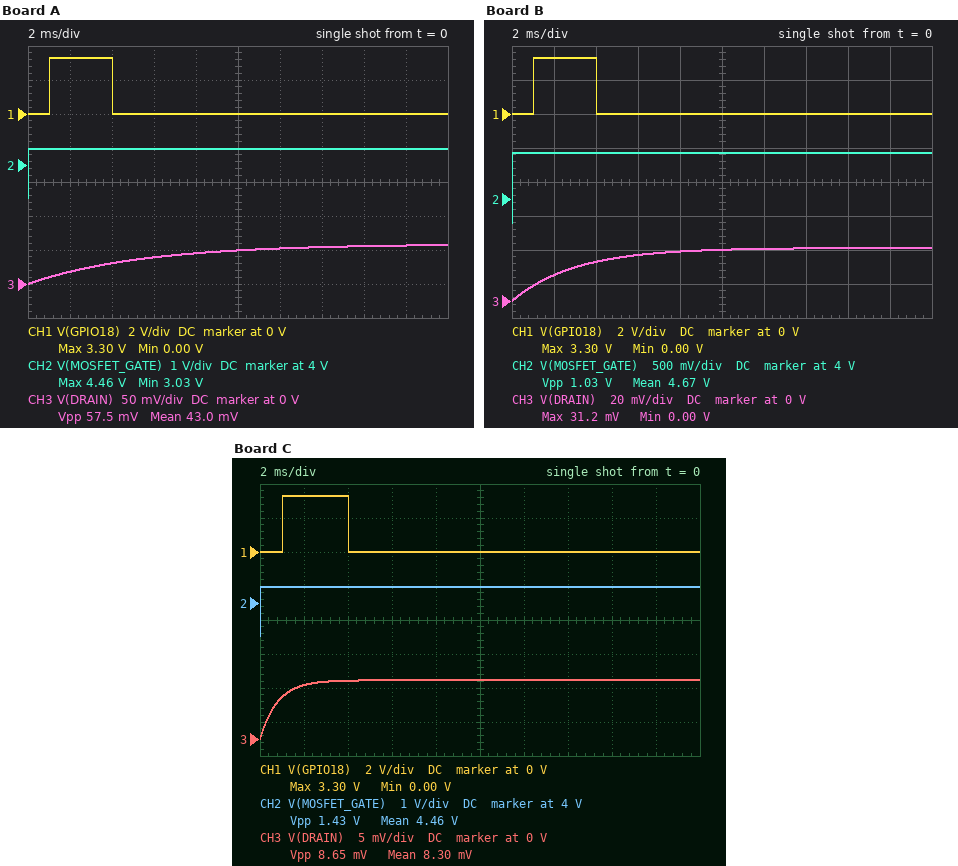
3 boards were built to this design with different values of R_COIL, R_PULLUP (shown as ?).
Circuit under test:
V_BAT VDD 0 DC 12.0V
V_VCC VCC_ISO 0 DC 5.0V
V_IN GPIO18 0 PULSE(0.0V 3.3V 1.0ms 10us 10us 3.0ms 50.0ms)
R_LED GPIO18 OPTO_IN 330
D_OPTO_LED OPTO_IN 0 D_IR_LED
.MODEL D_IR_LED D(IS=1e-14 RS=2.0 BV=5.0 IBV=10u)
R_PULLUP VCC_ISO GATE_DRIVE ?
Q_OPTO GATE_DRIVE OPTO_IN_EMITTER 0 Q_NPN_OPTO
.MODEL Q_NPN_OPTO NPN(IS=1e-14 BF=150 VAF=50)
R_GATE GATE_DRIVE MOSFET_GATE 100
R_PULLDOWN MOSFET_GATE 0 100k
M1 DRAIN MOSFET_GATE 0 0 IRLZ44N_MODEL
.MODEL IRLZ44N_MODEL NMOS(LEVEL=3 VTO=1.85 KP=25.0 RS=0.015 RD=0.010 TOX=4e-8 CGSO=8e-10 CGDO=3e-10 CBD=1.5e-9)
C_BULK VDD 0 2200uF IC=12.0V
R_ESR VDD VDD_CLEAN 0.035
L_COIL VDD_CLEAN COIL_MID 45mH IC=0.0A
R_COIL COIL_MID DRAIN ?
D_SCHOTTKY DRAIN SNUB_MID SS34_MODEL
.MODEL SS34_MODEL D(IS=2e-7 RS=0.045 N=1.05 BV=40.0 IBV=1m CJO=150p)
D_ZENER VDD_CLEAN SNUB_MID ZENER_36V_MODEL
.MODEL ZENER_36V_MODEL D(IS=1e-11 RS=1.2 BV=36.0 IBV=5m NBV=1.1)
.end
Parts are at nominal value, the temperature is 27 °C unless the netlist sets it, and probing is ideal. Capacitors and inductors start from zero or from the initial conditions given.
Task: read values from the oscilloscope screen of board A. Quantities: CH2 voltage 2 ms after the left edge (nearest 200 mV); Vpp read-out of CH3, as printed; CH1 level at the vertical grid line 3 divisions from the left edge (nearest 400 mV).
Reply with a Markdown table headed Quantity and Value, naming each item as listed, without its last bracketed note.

| Quantity | Value |
|---|---|
| CH2 voltage 2 ms after the left edge | 4.4 V |
| Vpp read-out of CH3, as printed | 57.5 mV |
| CH1 level at the vertical grid line 3 divisions from the left edge | 0 V |
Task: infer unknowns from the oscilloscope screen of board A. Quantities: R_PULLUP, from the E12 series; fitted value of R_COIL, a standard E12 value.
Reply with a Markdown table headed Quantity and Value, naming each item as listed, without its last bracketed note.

| Quantity | Value |
|---|---|
| R_PULLUP, from the E12 series | 12 kΩ |
| fitted value of R_COIL, a standard E12 value | 8.2 Ω |
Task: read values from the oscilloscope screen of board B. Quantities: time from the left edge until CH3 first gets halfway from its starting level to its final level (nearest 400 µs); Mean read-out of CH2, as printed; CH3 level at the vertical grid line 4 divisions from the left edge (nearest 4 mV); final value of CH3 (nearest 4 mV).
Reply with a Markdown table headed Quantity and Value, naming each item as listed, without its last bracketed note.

| Quantity | Value |
|---|---|
| time from the left edge until CH3 first gets halfway from its starting level to its final level | 2.0 ms |
| Mean read-out of CH2, as printed | 4.67 V |
| CH3 level at the vertical grid line 4 divisions from the left edge | 28 mV |
| final value of CH3 | 32 mV |
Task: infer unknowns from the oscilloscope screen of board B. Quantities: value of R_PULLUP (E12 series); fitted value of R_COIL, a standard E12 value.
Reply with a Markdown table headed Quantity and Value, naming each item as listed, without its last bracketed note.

| Quantity | Value |
|---|---|
| value of R_PULLUP | 6.8 kΩ |
| fitted value of R_COIL, a standard E12 value | 15 Ω |
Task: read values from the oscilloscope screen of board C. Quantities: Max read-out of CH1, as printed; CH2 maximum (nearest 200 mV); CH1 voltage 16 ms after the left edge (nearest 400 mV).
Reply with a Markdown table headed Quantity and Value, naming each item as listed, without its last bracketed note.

| Quantity | Value |
|---|---|
| Max read-out of CH1, as printed | 3.30 V |
| CH2 maximum | 4.4 V |
| CH1 voltage 16 ms after the left edge | 0 V |
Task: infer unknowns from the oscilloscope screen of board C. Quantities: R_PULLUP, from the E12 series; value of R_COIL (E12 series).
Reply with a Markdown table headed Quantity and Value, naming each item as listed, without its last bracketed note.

| Quantity | Value |
|---|---|
| R_PULLUP, from the E12 series | 12 kΩ |
| value of R_COIL | 56 Ω |
